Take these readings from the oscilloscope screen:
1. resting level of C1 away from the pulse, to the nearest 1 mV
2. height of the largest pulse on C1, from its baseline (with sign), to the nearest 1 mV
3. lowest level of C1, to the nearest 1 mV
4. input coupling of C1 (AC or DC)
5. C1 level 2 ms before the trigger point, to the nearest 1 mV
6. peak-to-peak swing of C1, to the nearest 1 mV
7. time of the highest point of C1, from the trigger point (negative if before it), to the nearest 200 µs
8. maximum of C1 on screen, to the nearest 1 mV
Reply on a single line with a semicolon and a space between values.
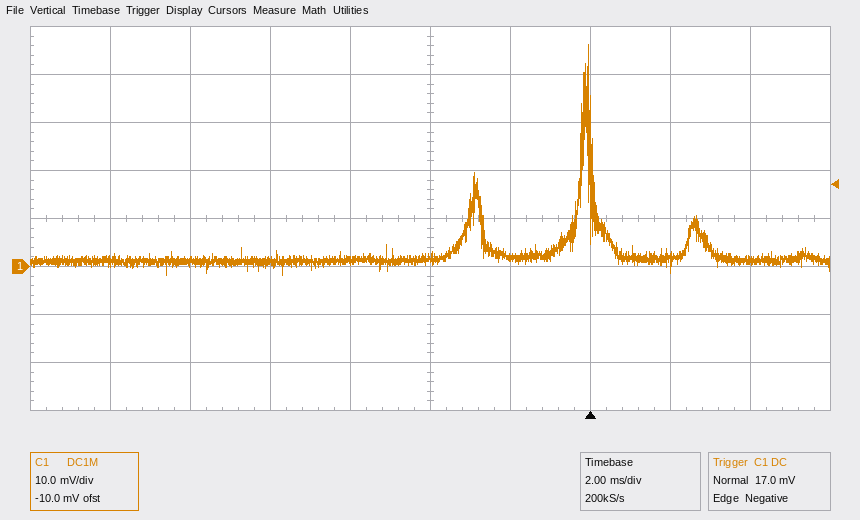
1 mV; +45 mV; -2 mV; DC; 2 mV; 48 mV; 0.0 ms; 46 mV
